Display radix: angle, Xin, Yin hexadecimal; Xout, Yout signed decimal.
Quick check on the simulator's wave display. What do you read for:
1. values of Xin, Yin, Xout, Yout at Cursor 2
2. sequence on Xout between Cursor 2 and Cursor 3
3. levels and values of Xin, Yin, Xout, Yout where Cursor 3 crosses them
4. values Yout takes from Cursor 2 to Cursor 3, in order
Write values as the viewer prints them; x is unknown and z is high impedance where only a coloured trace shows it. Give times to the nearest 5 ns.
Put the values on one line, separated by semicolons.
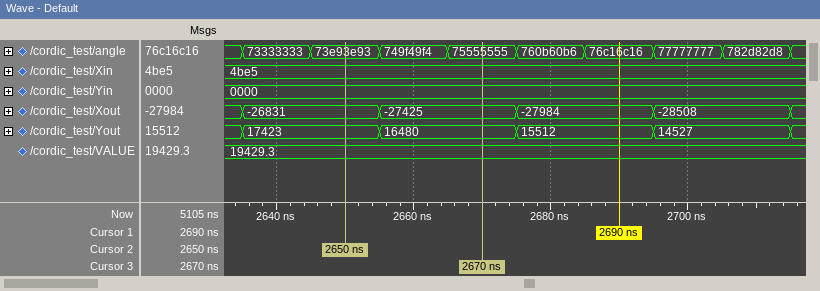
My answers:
Xin=4be5, Yin=0000, Xout=-26831, Yout=17423; -26831, -27425; Xin=4be5, Yin=0000, Xout=-27425, Yout=16480; 17423, 16480
